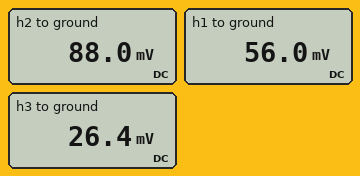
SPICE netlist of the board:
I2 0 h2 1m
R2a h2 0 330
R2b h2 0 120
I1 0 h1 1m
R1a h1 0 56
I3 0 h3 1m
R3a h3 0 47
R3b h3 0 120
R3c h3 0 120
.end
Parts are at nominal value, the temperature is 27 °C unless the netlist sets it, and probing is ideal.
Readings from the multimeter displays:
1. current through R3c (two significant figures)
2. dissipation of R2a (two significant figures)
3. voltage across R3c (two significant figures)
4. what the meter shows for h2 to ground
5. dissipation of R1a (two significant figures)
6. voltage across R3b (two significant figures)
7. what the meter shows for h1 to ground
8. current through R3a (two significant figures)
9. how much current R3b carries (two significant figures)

220 µA
23 µW
26 mV
88.0 mV
56 µW
26 mV
56.0 mV
560 µA
220 µA
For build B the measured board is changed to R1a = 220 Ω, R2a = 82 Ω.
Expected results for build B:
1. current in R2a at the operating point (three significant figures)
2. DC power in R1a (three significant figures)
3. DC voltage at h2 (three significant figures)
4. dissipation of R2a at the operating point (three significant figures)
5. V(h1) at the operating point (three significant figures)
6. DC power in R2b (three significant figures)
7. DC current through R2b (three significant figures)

594 µA
220 µW
48.7 mV
28.9 µW
220 mV
19.8 µW
406 µA
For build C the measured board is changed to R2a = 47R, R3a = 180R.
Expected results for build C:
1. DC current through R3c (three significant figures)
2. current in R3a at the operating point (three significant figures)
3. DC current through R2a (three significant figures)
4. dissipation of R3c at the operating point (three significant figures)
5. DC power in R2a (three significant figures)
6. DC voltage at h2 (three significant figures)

375 µA
250 µA
719 µA
16.9 µW
24.3 µW
33.8 mV
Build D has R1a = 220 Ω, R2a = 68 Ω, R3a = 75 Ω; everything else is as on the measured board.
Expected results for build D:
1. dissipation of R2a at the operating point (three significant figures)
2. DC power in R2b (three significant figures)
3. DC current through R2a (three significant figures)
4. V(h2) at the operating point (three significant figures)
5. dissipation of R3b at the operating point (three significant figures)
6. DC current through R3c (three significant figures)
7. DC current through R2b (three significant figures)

27.7 µW
15.7 µW
638 µA
43.4 mV
9.26 µW
278 µA
362 µA
